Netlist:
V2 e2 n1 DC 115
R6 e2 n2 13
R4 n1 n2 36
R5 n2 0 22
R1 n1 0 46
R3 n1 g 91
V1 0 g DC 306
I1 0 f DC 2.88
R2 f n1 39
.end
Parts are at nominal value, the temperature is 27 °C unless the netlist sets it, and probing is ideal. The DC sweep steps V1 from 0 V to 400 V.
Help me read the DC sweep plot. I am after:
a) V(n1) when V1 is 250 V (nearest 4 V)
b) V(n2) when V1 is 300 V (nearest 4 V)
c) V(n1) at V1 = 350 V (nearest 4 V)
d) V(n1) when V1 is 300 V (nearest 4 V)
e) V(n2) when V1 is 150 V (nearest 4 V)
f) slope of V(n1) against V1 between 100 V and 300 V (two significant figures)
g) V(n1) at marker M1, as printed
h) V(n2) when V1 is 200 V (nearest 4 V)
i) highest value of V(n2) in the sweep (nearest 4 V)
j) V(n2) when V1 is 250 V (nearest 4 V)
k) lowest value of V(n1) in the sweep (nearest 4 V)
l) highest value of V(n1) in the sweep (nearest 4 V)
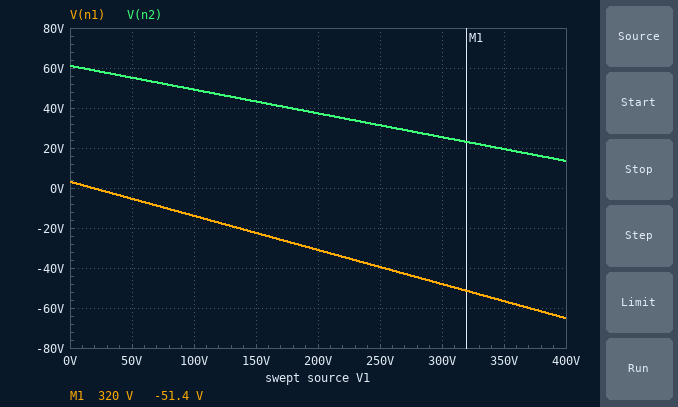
-40 V
24 V
-56 V
-48 V
44 V
-0.17 V/V
-51.4 V
36 V
60 V
32 V
-64 V
4 V
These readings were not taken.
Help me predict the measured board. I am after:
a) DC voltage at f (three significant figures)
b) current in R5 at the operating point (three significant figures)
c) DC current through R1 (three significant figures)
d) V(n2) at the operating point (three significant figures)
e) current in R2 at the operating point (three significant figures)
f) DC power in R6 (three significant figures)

63.3 V
1.12 A
1.07 A
24.7 V
2.88 A
131 W
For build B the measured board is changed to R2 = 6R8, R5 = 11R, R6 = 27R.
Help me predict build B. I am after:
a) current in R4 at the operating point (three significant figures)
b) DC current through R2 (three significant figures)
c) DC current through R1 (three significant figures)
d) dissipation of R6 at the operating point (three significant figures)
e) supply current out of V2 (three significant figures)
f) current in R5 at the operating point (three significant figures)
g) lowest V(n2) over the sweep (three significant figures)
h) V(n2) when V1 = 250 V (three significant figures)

1.44 A
2.88 A
915 mA
147 W
2.34 A
894 mA
3.75 V
13.5 V
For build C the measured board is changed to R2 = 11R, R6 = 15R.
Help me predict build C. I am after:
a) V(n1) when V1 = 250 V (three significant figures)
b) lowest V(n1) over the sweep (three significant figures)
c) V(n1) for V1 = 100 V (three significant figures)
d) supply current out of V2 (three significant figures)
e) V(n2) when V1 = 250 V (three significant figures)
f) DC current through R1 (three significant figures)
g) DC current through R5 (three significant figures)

-37.2 V
-63.2 V
-11.2 V
3.00 A
29.7 V
1.02 A
1.05 A
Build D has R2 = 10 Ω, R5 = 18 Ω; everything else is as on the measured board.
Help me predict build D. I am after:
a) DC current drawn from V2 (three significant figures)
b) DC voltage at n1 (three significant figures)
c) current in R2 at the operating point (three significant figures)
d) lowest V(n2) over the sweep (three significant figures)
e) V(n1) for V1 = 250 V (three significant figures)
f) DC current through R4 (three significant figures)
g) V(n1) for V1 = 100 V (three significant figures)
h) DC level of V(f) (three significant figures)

3.23 A
-51.4 V
2.88 A
11.8 V
-42.5 V
2.03 A
-18.6 V
-22.6 V
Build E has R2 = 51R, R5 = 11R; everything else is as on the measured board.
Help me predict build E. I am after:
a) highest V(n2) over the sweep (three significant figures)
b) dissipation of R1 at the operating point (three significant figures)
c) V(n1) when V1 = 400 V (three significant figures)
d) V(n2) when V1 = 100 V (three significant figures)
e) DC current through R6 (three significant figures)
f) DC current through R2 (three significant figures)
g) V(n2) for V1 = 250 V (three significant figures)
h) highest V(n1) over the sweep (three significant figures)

37.1 V
69.3 W
-69.1 V
29.9 V
3.35 A
2.88 A
19.1 V
-15.1 V
